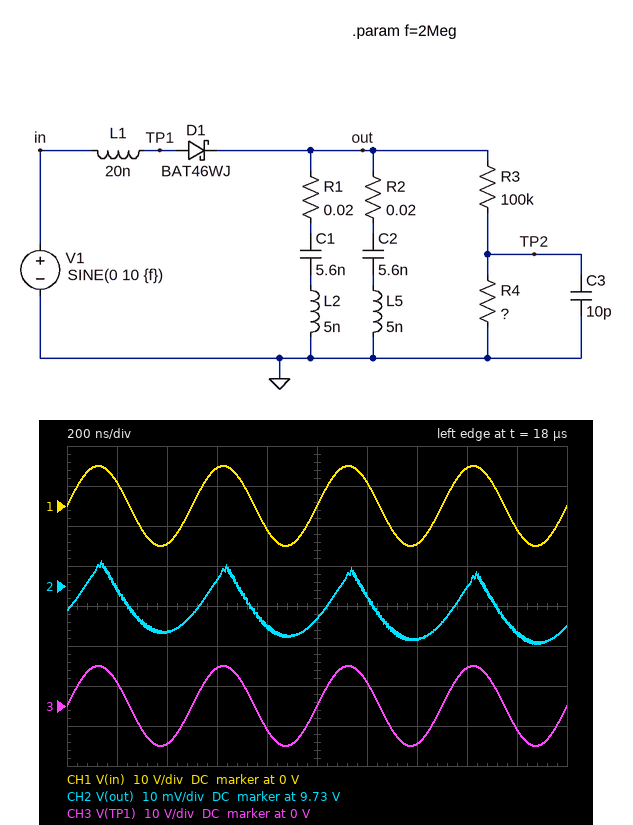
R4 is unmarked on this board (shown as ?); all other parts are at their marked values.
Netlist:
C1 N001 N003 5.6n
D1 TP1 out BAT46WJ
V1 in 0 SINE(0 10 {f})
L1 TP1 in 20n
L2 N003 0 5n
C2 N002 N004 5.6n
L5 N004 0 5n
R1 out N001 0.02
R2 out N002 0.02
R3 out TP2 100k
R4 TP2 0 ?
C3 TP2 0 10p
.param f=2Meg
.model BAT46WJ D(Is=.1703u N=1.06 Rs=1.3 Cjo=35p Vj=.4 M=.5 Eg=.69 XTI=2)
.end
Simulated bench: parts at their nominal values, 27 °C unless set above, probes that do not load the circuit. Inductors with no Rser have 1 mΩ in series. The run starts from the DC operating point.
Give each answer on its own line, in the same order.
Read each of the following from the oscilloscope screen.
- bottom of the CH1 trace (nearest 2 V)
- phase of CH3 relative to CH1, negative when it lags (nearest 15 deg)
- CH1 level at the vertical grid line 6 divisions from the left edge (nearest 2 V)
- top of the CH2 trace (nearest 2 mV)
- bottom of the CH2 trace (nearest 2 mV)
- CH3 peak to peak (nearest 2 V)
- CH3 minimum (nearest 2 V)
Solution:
-10 V
0 deg
6 V
9.736 V
9.716 V
20 V
-10 V
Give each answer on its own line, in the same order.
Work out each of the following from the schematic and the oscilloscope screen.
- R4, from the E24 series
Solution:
27 kΩ
